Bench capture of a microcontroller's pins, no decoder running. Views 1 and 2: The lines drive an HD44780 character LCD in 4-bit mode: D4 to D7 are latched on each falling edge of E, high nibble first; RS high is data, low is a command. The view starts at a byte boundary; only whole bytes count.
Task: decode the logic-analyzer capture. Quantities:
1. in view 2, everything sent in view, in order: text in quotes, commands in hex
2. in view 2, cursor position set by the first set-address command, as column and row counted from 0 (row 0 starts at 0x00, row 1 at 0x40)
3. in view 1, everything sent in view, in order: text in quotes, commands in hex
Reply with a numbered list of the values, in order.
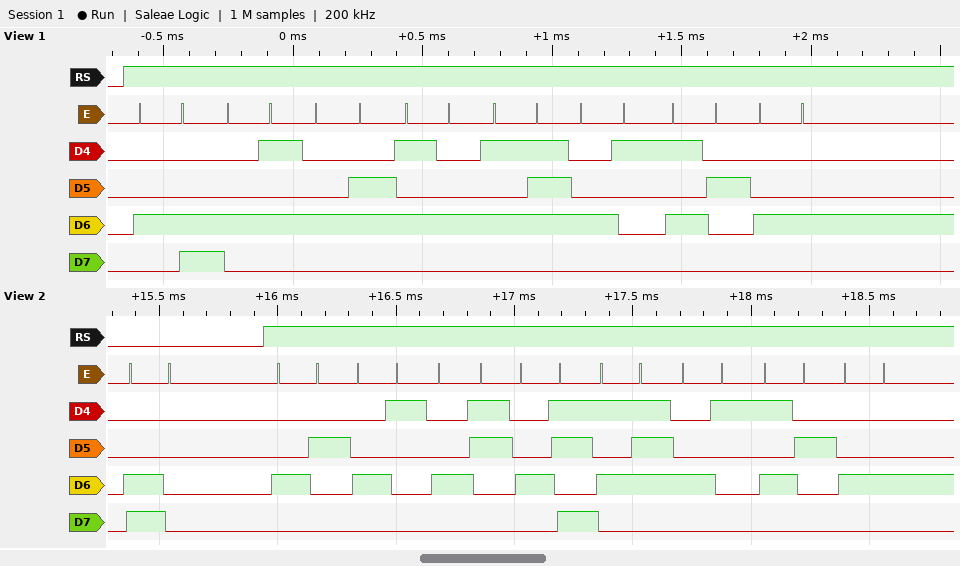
1. 0xC0 "BACKWARD"
2. column 0, row 1
3. "LEFTWARD"
